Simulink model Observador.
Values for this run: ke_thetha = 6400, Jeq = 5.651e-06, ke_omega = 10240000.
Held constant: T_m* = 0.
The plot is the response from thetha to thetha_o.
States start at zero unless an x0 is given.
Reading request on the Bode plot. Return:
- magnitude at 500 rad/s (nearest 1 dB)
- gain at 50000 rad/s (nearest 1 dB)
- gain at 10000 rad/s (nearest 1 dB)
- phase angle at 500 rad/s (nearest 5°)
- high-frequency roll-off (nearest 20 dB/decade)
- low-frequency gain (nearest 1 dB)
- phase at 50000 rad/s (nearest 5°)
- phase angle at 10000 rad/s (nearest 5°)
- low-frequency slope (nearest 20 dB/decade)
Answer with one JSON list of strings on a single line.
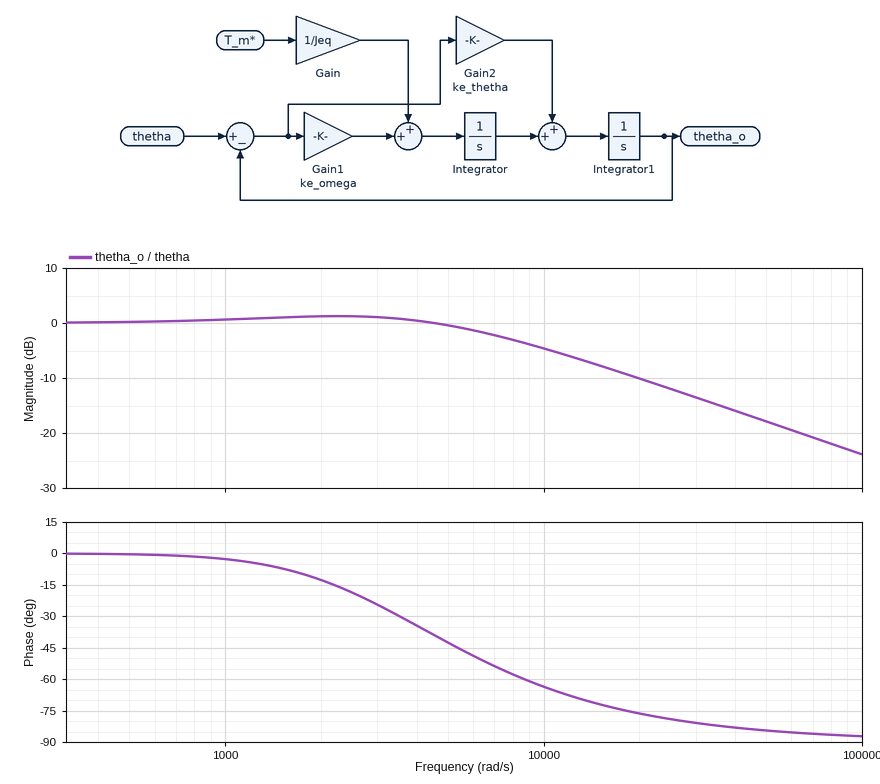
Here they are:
["0 dB", "-18 dB", "-5 dB", "0°", "-20 dB/decade", "0 dB", "-85°", "-65°", "0 dB/decade"]
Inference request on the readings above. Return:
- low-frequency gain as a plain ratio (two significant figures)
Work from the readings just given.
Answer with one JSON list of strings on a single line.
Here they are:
["1.0"]
